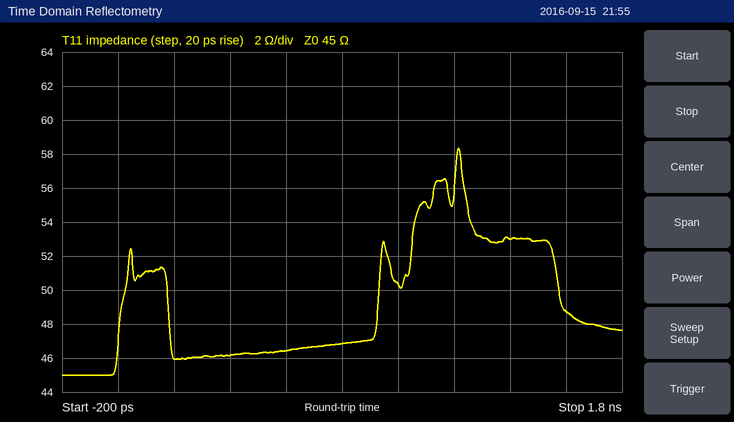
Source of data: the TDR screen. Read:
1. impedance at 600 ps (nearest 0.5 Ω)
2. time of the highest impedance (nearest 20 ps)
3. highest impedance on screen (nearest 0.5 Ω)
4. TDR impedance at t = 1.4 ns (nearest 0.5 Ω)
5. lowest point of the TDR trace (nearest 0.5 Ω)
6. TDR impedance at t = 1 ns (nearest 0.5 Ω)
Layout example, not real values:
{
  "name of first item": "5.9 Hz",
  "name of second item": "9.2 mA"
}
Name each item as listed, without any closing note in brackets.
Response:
{
  "impedance at 600 ps": "46.5 Ω",
  "time of the highest impedance": "1.22 ns",
  "highest impedance on screen": "58.5 Ω",
  "TDR impedance at t = 1.4 ns": "53.0 Ω",
  "lowest point of the TDR trace": "45.0 Ω",
  "TDR impedance at t = 1 ns": "50.5 Ω"
}
